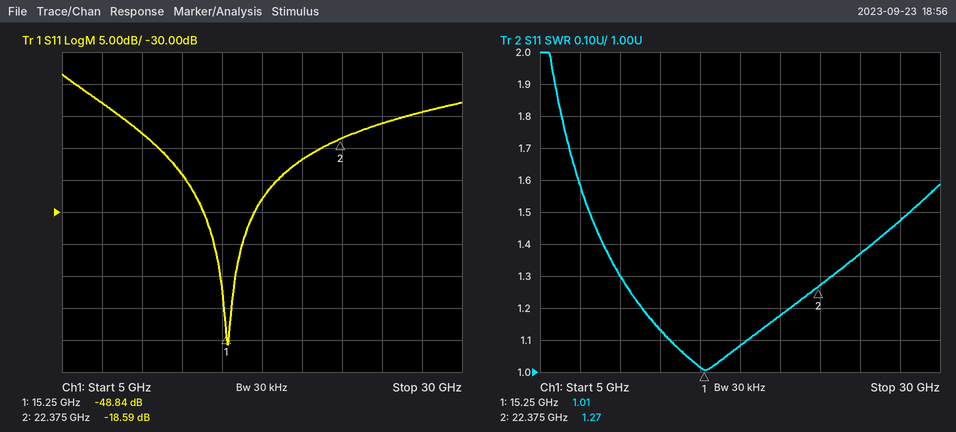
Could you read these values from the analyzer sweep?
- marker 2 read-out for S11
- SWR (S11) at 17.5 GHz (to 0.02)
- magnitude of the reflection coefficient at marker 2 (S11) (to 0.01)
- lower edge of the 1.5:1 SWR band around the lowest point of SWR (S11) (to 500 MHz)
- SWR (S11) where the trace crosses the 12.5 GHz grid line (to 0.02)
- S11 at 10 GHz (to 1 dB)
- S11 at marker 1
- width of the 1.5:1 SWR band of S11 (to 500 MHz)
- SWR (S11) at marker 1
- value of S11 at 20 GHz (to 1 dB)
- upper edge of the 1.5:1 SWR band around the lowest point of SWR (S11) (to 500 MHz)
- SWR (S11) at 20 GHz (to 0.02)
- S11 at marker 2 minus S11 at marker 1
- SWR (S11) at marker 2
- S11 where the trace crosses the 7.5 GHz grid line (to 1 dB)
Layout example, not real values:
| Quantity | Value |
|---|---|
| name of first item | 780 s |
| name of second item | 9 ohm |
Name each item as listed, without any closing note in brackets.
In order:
| Quantity | Value |
|---|---|
| marker 2 read-out for S11 | -18.59 dB |
| SWR (S11) at 17.5 GHz | 1.08 |
| magnitude of the reflection coefficient at marker 2 (S11) | 0.12 |
| lower edge of the 1.5:1 SWR band around the lowest point of SWR (S11) | 8.0 GHz |
| SWR (S11) where the trace crosses the 12.5 GHz grid line | 1.14 |
| S11 at 10 GHz | -18 dB |
| S11 at marker 1 | -48.84 dB |
| width of the 1.5:1 SWR band of S11 | 20.0 GHz |
| SWR (S11) at marker 1 | 1.01 |
| value of S11 at 20 GHz | -22 dB |
| upper edge of the 1.5:1 SWR band around the lowest point of SWR (S11) | 28.0 GHz |
| SWR (S11) at 20 GHz | 1.18 |
| S11 at marker 2 minus S11 at marker 1 | 30.25 dB |
| SWR (S11) at marker 2 | 1.27 |
| S11 where the trace crosses the 7.5 GHz grid line | -13 dB |
